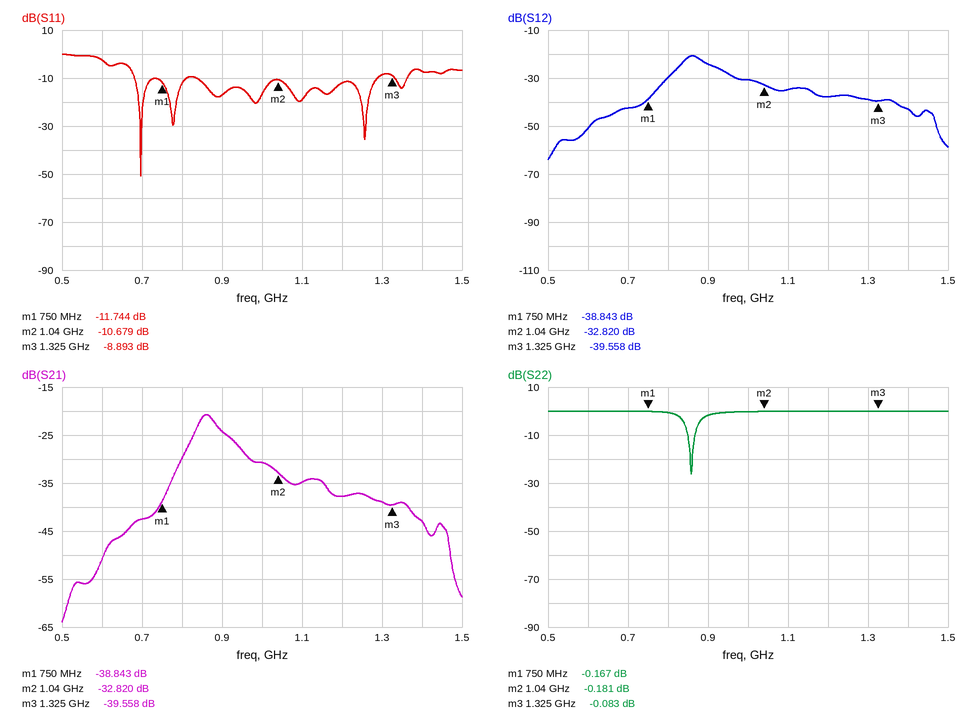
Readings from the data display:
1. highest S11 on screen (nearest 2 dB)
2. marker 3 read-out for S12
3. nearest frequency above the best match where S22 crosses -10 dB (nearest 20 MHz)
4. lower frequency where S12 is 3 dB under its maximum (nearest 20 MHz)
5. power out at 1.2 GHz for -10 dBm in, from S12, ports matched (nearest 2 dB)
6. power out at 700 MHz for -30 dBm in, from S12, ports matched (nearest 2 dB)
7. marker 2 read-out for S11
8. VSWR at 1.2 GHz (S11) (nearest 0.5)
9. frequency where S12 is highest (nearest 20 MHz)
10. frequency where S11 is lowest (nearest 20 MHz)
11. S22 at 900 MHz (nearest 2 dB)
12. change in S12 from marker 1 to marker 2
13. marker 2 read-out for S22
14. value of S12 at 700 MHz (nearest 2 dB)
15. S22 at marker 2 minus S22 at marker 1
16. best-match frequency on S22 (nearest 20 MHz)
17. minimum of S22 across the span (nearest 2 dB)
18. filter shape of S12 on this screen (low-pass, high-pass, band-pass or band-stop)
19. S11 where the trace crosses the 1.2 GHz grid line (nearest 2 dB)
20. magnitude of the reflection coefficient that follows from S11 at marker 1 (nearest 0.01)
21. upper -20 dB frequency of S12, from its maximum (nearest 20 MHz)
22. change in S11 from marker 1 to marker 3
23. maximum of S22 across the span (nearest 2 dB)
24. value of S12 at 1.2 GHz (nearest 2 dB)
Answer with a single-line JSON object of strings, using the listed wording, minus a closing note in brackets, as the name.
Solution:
{"highest S11 on screen": "0 dB", "marker 3 read-out for S12": "-39.558 dB", "nearest frequency above the best match where S22 crosses -10 dB": "860 MHz", "lower frequency where S12 is 3 dB under its maximum": "840 MHz", "power out at 1.2 GHz for -10 dBm in, from S12, ports matched": "-48 dBm", "power out at 700 MHz for -30 dBm in, from S12, ports matched": "-72 dBm", "marker 2 read-out for S11": "-10.679 dB", "VSWR at 1.2 GHz (S11)": "1.5", "frequency where S12 is highest": "860 MHz", "frequency where S11 is lowest": "700 MHz", "S22 at 900 MHz": "-2 dB", "change in S12 from marker 1 to marker 2": "6.023 dB", "marker 2 read-out for S22": "-0.181 dB", "value of S12 at 700 MHz": "-42 dB", "S22 at marker 2 minus S22 at marker 1": "-0.014 dB", "best-match frequency on S22": "860 MHz", "minimum of S22 across the span": "-26 dB", "filter shape of S12 on this screen": "band-pass", "S11 where the trace crosses the 1.2 GHz grid line": "-12 dB", "magnitude of the reflection coefficient that follows from S11 at marker 1": "0.26", "upper -20 dB frequency of S12, from its maximum": "1.38 GHz", "change in S11 from marker 1 to marker 3": "2.851 dB", "maximum of S22 across the span": "0 dB", "value of S12 at 1.2 GHz": "-38 dB"}
